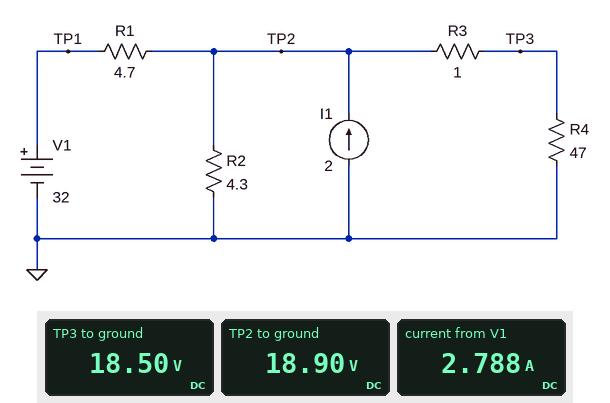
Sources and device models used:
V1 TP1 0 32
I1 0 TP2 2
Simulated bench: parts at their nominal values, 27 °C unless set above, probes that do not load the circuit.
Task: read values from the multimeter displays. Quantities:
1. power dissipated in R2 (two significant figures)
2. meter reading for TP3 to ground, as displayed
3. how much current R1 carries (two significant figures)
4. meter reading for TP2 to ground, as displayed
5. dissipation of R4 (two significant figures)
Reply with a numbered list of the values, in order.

1. 83 W
2. 18.50 V
3. 2.8 A
4. 18.90 V
5. 7.3 W
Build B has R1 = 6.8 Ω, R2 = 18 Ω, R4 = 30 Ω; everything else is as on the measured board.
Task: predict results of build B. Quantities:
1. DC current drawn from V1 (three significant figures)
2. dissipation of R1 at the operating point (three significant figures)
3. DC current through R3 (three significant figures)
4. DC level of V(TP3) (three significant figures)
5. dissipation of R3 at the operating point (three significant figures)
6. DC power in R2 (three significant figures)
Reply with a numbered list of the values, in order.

1. 507 mA
2. 1.75 W
3. 921 mA
4. 27.6 V
5. 848 mW
6. 45.3 W
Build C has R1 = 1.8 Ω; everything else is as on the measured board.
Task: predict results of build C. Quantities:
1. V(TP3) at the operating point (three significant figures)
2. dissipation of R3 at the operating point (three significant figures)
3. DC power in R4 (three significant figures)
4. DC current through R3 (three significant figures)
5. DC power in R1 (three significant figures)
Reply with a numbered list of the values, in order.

1. 23.9 V
2. 259 mW
3. 12.2 W
4. 509 mA
5. 31.7 W
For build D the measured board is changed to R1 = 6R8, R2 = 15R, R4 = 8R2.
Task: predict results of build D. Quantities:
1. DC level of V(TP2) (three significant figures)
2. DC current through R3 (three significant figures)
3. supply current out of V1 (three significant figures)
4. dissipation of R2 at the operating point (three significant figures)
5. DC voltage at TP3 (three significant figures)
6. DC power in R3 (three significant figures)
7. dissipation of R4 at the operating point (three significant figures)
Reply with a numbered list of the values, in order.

1. 20.8 V
2. 2.26 A
3. 1.65 A
4. 28.8 W
5. 18.5 V
6. 5.11 W
7. 41.9 W
